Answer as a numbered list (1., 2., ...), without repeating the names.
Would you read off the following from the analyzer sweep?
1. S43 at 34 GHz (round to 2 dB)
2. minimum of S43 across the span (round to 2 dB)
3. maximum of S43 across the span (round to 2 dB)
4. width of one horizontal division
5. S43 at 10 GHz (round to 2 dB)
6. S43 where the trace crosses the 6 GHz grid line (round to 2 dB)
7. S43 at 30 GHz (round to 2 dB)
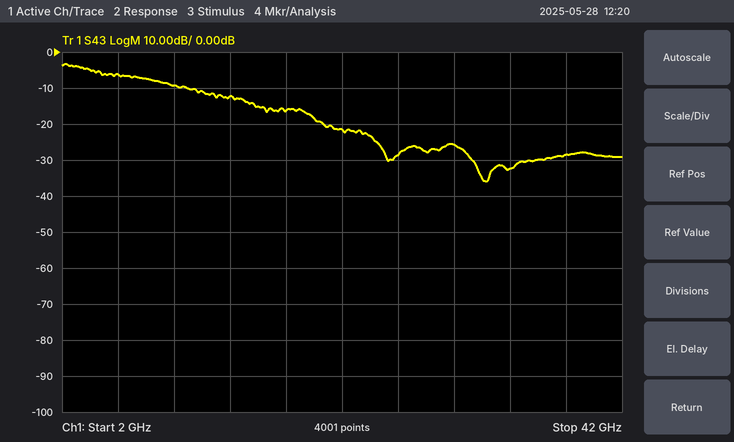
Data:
1. -32 dB
2. -36 dB
3. -4 dB
4. 4 GHz
5. -10 dB
6. -6 dB
7. -26 dB
